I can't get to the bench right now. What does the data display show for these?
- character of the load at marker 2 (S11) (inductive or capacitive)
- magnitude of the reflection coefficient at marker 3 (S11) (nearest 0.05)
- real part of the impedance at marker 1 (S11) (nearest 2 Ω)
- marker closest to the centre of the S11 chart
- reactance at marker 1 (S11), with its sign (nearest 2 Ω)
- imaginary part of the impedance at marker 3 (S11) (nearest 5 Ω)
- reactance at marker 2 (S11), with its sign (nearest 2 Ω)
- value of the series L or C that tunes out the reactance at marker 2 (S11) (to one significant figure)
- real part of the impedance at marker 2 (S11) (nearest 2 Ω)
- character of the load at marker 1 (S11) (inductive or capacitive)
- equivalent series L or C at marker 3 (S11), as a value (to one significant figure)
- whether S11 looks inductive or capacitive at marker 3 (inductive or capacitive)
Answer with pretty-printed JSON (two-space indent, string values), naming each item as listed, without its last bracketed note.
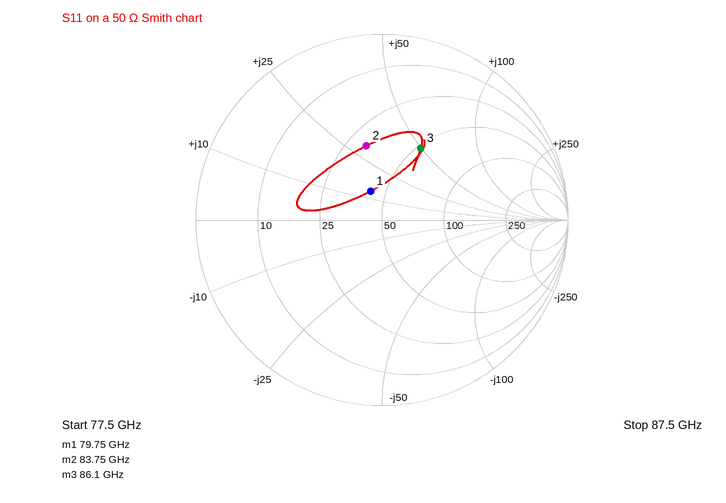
{
  "character of the load at marker 2 (S11)": "inductive",
  "magnitude of the reflection coefficient at marker 3 (S11)": "0.45",
  "real part of the impedance at marker 1 (S11)": "42 Ω",
  "marker closest to the centre of the S11 chart": "marker 1",
  "reactance at marker 1 (S11), with its sign": "+14 Ω",
  "imaginary part of the impedance at marker 3 (S11)": "+50 Ω",
  "reactance at marker 2 (S11), with its sign": "+30 Ω",
  "value of the series L or C that tunes out the reactance at marker 2 (S11)": "60 fF",
  "real part of the impedance at marker 2 (S11)": "32 Ω",
  "character of the load at marker 1 (S11)": "inductive",
  "equivalent series L or C at marker 3 (S11), as a value": "90 pH",
  "whether S11 looks inductive or capacitive at marker 3": "inductive"
}
